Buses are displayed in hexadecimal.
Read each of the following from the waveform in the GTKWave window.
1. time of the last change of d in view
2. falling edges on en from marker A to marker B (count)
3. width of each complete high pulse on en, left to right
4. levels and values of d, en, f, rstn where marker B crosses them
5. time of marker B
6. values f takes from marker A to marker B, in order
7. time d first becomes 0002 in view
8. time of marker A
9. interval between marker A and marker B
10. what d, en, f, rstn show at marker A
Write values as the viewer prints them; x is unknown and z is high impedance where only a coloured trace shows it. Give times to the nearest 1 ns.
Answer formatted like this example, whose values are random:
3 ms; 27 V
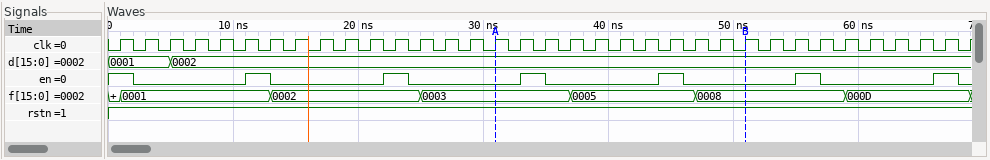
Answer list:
5 ns; 2; 2 ns, 2 ns, 2 ns, 2 ns, 2 ns, 2 ns; d=0002, en=0, f=0008, rstn=1; 51 ns; 0003, 0005, 0008; 5 ns; 31 ns; 20 ns; d=0002, en=0, f=0003, rstn=1
